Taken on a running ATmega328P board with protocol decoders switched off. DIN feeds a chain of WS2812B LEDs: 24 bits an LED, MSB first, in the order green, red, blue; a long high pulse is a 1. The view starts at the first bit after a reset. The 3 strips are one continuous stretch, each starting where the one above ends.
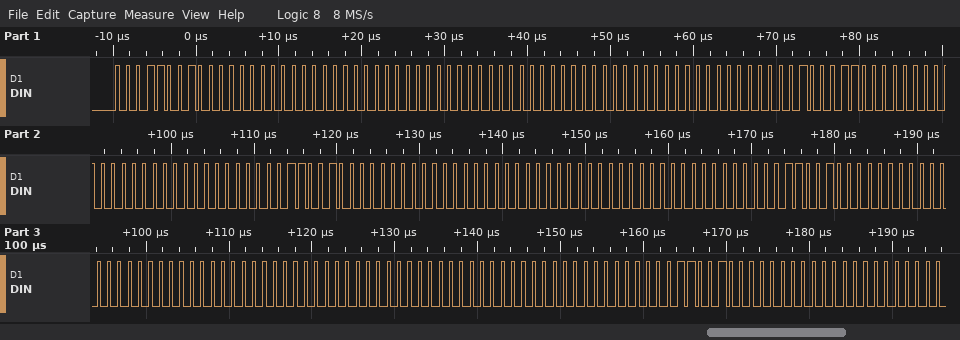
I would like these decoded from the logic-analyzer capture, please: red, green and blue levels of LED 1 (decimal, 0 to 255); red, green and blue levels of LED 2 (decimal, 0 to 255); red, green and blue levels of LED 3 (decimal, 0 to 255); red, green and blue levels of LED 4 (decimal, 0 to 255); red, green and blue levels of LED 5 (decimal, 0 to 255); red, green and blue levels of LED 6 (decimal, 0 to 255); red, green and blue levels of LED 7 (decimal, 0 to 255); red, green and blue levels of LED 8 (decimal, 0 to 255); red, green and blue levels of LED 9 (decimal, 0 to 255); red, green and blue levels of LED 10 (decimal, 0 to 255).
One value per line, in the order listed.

0, 25, 0
0, 0, 0
0, 0, 35
0, 0, 0
0, 25, 0
0, 0, 0
0, 25, 0
0, 0, 0
0, 0, 0
0, 25, 0
